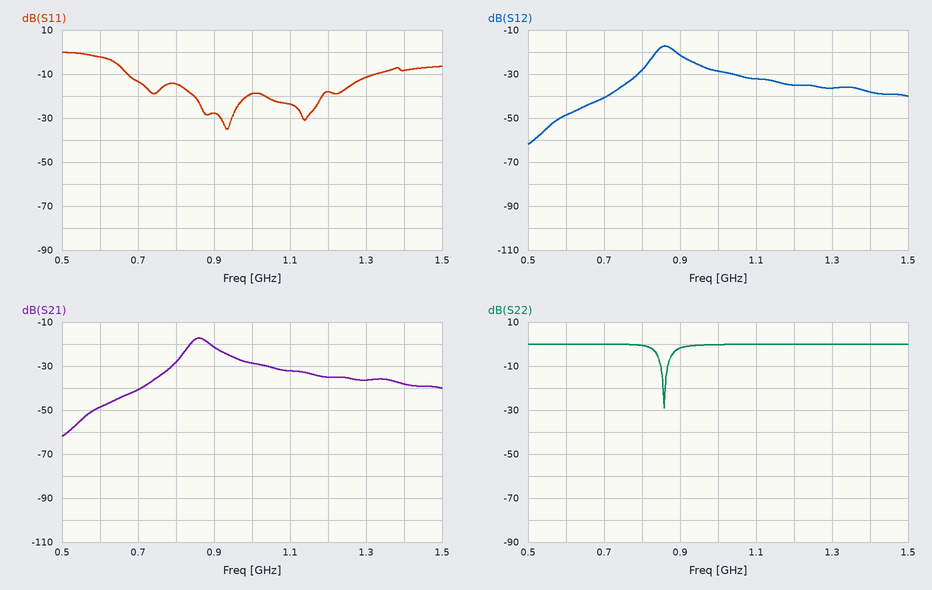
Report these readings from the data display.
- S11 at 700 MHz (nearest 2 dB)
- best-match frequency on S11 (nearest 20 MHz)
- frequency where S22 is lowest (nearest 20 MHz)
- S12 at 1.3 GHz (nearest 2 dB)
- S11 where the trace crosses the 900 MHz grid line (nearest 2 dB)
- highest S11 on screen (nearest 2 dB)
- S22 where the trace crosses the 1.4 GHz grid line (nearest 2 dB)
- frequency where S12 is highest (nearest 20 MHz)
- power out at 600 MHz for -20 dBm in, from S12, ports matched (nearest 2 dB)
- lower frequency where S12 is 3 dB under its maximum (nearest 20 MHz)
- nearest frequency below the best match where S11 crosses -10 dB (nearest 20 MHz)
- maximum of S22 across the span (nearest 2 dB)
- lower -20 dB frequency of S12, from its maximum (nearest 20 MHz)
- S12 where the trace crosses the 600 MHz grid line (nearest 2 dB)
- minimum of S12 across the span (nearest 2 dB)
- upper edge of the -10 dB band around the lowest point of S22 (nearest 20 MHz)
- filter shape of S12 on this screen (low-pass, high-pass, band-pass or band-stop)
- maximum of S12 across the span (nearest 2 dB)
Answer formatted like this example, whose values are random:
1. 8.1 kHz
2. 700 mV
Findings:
1. -14 dB
2. 940 MHz
3. 860 MHz
4. -36 dB
5. -28 dB
6. 0 dB
7. 0 dB
8. 860 MHz
9. -68 dBm
10. 840 MHz
11. 680 MHz
12. 0 dB
13. 740 MHz
14. -48 dB
15. -62 dB
16. 860 MHz
17. band-pass
18. -18 dB
